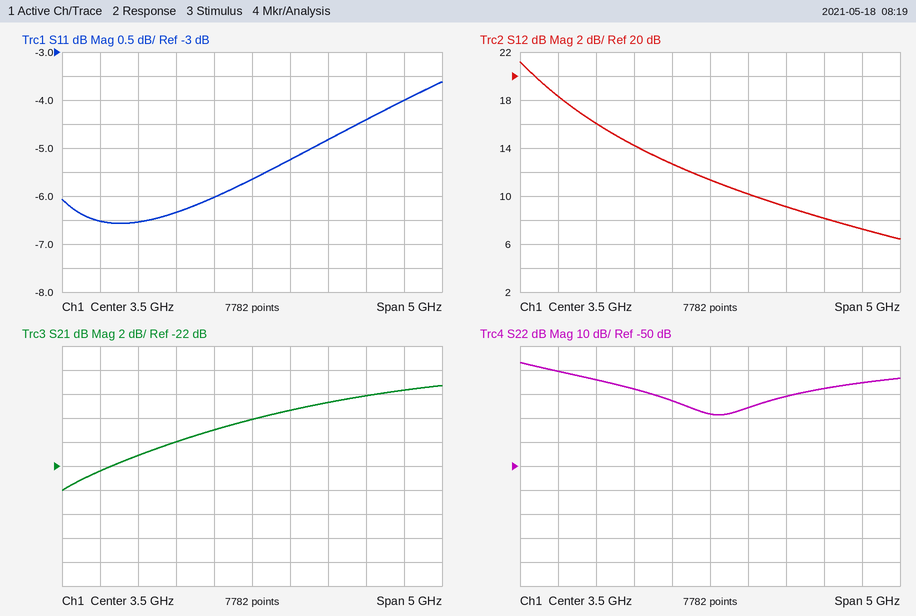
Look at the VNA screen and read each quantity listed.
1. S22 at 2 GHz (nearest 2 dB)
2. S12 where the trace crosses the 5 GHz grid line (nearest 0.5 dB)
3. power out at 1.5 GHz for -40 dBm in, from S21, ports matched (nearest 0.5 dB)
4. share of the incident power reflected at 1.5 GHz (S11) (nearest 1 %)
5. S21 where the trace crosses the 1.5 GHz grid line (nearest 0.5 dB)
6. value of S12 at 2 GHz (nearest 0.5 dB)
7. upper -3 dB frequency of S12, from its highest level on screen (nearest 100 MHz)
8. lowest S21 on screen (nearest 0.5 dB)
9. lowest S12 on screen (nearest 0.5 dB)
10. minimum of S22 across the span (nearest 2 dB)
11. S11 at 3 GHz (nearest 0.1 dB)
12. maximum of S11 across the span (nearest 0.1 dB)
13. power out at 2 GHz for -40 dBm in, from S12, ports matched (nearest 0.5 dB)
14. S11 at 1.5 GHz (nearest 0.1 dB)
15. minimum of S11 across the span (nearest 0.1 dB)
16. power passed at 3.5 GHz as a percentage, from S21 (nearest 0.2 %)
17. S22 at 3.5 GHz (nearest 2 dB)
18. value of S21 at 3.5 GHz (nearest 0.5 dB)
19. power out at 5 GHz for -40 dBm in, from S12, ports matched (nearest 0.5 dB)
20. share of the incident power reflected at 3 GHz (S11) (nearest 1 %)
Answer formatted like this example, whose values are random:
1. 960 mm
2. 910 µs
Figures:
1. -14 dB
2. 8.0 dB
3. -62.5 dBm
4. 22 %
5. -22.5 dB
6. 16.0 dB
7. 1.5 GHz
8. -24.0 dB
9. 6.5 dB
10. -28 dB
11. -6.0 dB
12. -3.6 dB
13. -24.0 dBm
14. -6.5 dB
15. -6.6 dB
16. 1.6 %
17. -28 dB
18. -18.0 dB
19. -32.0 dBm
20. 25 %
